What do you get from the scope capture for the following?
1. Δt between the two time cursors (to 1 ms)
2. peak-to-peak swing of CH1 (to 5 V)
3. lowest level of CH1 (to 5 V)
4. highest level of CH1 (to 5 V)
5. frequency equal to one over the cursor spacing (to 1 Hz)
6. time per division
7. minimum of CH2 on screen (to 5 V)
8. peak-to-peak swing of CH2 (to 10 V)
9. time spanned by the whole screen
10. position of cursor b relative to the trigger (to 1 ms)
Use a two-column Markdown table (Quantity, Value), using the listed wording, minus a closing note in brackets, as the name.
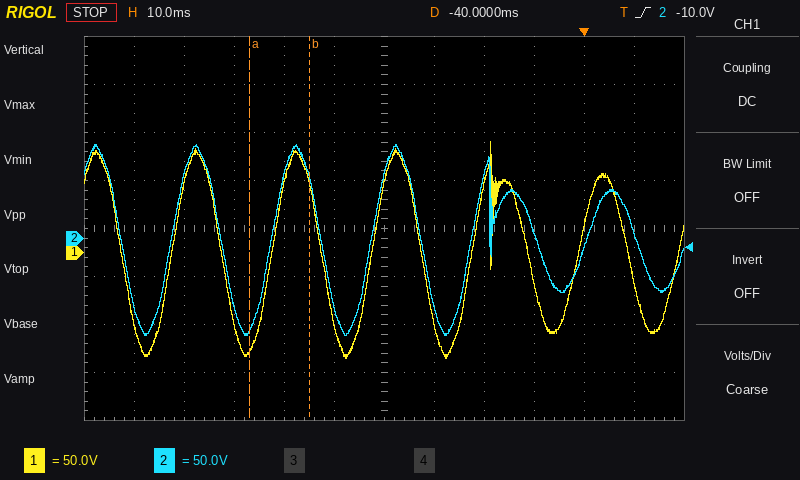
| Quantity | Value |
|---|---|
| Δt between the two time cursors | 12 ms |
| peak-to-peak swing of CH1 | 225 V |
| lowest level of CH1 | -110 V |
| highest level of CH1 | 115 V |
| frequency equal to one over the cursor spacing | 83 Hz |
| time per division | 10 ms |
| minimum of CH2 on screen | -100 V |
| peak-to-peak swing of CH2 | 200 V |
| time spanned by the whole screen | 120 ms |
| position of cursor b relative to the trigger | -55 ms |
